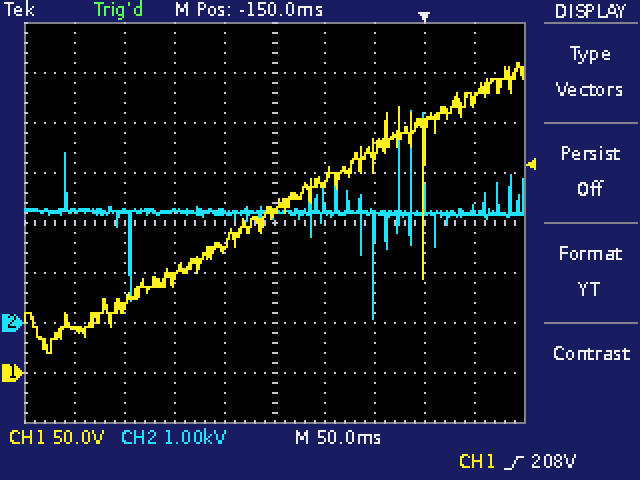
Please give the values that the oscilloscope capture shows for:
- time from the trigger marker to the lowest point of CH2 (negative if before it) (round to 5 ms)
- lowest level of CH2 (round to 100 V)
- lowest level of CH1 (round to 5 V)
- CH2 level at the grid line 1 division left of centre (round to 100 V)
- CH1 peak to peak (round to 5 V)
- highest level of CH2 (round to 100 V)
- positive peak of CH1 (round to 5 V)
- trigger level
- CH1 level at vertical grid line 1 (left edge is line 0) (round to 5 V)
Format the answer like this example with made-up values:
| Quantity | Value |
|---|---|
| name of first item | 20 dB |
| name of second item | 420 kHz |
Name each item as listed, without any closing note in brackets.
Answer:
| Quantity | Value |
|---|---|
| time from the trigger marker to the lowest point of CH2 (negative if before it) | -50 ms |
| lowest level of CH2 | 100 V |
| lowest level of CH1 | 20 V |
| CH2 level at the grid line 1 division left of centre | 2.2 kV |
| CH1 peak to peak | 290 V |
| highest level of CH2 | 4.2 kV |
| positive peak of CH1 | 310 V |
| trigger level | 208 V |
| CH1 level at vertical grid line 1 (left edge is line 0) | 45 V |
